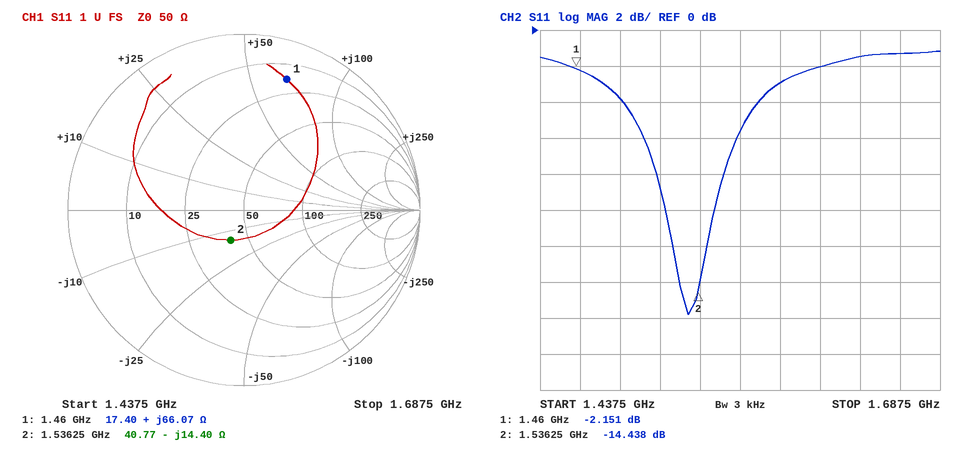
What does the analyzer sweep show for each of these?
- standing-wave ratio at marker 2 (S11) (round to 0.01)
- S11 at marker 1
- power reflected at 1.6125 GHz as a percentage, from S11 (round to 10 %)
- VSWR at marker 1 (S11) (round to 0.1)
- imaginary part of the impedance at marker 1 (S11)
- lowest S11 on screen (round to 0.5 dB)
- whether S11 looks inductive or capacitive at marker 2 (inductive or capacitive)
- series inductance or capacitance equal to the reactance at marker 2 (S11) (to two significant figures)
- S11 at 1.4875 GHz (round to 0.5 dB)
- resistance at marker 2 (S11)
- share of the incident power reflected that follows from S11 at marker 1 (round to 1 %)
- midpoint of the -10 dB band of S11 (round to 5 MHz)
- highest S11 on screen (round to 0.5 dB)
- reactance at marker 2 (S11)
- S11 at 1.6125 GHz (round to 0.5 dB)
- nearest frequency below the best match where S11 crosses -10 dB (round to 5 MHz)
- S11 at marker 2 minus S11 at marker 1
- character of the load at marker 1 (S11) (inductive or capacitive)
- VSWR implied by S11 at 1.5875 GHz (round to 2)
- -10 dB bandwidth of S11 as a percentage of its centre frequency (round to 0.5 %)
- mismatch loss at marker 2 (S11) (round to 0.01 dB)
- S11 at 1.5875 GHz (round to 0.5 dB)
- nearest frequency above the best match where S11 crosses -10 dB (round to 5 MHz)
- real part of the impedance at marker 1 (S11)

1.46
-2.151 dB
60 %
8.1
+66.07 Ω
-16.0 dB
capacitive
7.2 pF
-4.0 dB
40.77 Ω
61 %
1.530 GHz
-1.0 dB
-14.40 Ω
-2.0 dB
1.515 GHz
-12.287 dB
inductive
6
2.0 %
0.16 dB
-3.0 dB
1.545 GHz
17.40 Ω
